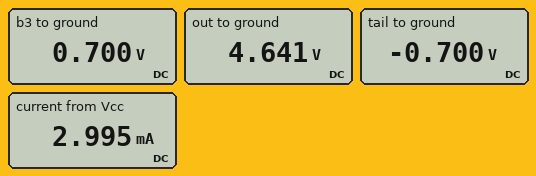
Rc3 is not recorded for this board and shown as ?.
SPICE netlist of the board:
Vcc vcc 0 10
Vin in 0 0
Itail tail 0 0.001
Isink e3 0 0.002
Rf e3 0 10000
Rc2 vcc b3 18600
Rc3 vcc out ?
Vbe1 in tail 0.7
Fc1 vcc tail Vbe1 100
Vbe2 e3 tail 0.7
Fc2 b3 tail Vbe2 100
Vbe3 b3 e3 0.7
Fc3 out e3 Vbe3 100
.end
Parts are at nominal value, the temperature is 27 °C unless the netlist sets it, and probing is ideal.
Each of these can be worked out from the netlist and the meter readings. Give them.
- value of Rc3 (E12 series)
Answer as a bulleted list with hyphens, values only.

- 2.7 kΩ
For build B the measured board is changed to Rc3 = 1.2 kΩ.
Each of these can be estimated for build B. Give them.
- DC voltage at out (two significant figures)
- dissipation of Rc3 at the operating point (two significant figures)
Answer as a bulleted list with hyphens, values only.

- 7.6 V
- 4.7 mW
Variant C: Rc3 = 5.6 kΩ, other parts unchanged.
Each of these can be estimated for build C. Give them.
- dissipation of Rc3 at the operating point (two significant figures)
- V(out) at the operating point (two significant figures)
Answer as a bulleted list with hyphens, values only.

- 22 mW
- -1.1 V
